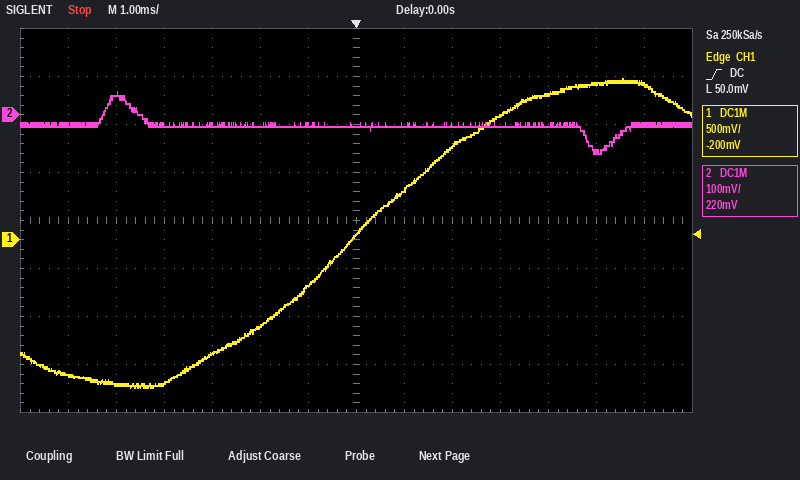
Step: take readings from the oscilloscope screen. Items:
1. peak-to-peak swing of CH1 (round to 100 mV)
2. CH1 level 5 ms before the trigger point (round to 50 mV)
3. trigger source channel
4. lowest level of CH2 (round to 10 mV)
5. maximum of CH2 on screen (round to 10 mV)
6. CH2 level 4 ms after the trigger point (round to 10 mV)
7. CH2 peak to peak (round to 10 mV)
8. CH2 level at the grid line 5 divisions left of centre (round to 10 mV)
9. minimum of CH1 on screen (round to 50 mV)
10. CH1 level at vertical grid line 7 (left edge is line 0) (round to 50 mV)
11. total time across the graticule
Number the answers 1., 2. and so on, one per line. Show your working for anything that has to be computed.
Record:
1. 3.20 V
2. -1.50 V
3. CH1
4. -80 mV
5. 50 mV
6. -20 mV
7. 50 mV − (-80 mV) = 130 mV
8. 40 mV
9. -1.55 V
10. 50 mV
11. 14 ms
